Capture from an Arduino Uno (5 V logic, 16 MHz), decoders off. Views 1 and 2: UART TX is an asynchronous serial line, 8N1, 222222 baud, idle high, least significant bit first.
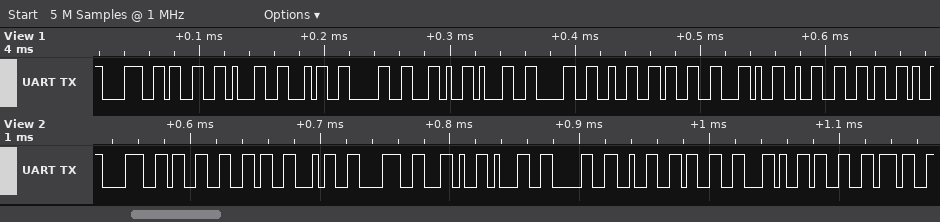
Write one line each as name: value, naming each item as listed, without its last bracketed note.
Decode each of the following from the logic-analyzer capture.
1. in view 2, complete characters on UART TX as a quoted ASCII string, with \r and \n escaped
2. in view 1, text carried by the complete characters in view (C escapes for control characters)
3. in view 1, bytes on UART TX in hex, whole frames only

in view 2, complete characters on UART TX as a quoted ASCII string, with \r and \n escaped: "83648,1023,37"
in view 1, text carried by the complete characters in view: "83140,1023,26"
in view 1, bytes on UART TX in hex, whole frames only: 0x38 0x33 0x31 0x34 0x30 0x2C 0x31 0x30 0x32 0x33 0x2C 0x32 0x36
